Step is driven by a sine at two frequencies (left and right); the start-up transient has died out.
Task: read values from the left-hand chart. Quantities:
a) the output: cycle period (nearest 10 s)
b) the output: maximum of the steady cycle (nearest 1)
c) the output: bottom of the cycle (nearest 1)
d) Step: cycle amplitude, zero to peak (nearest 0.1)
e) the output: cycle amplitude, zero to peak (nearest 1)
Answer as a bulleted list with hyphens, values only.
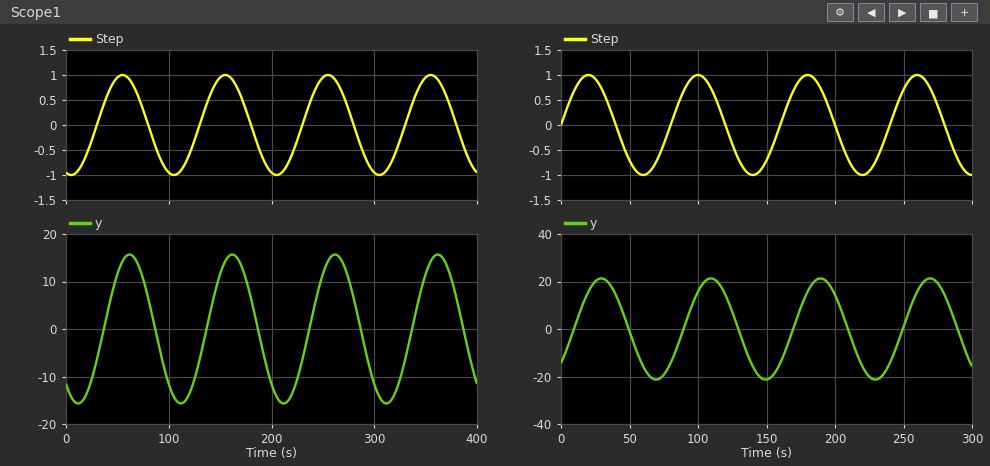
- 100 s
- 16
- -16
- 1.0
- 16
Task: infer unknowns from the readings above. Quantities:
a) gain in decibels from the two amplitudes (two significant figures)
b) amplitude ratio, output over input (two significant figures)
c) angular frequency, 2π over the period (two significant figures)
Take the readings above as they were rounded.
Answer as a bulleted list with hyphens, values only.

- 24 dB
- 16
- 0.063 rad/s
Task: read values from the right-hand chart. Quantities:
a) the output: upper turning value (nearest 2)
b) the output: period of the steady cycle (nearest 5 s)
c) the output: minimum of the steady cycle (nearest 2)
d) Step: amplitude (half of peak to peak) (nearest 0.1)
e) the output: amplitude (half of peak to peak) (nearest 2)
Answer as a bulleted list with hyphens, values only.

- 22
- 80 s
- -22
- 1.0
- 22
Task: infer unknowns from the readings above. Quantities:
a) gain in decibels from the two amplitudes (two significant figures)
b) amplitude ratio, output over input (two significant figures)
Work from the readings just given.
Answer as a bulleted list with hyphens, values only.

- 27 dB
- 22
